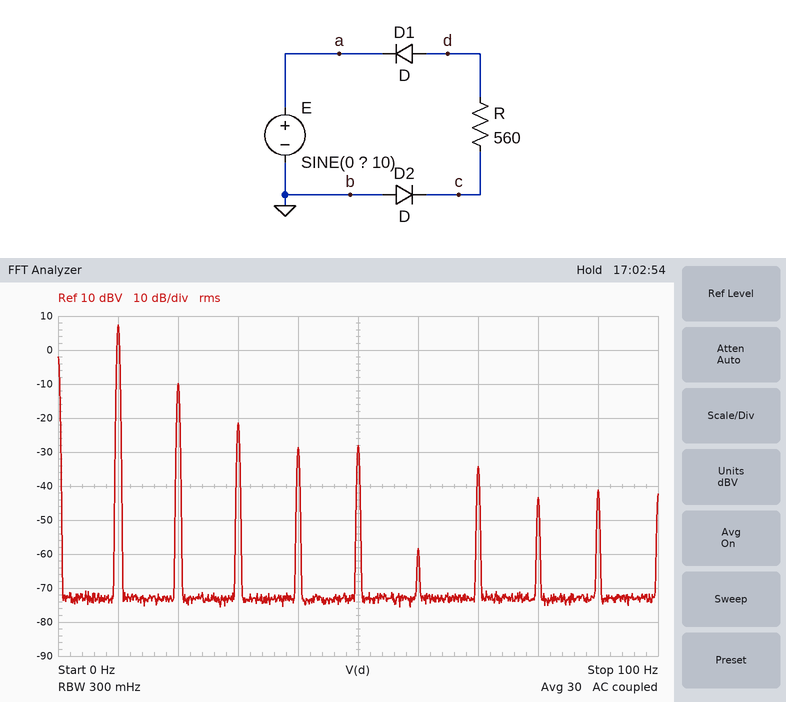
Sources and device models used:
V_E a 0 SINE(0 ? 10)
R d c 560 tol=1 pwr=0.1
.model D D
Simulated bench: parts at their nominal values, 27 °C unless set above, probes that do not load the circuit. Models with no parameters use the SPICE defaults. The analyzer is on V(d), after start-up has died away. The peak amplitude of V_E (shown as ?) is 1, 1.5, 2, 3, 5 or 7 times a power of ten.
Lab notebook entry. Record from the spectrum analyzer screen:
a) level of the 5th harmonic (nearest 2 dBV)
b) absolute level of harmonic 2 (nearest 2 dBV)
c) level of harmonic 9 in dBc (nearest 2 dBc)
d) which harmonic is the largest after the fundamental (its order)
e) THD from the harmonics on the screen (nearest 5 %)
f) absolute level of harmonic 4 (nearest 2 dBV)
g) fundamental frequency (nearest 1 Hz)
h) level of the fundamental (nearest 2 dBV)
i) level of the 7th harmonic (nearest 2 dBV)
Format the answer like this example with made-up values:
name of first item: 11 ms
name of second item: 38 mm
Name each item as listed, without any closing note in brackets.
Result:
level of the 5th harmonic: -28 dBV
absolute level of harmonic 2: -10 dBV
level of harmonic 9 in dBc: -48 dBc
which harmonic is the largest after the fundamental: 2
THD from the harmonics on the screen: 15 %
absolute level of harmonic 4: -28 dBV
fundamental frequency: 10 Hz
level of the fundamental: 8 dBV
level of the 7th harmonic: -34 dBV
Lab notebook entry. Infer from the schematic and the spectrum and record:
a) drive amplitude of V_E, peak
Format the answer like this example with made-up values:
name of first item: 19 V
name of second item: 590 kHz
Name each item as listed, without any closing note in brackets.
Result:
drive amplitude of V_E, peak: 5 V
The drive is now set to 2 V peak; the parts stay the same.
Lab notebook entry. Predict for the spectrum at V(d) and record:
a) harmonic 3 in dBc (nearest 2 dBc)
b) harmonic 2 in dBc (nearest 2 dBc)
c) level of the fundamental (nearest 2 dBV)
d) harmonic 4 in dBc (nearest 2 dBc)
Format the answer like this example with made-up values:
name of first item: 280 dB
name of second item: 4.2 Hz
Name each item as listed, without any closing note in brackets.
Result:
harmonic 3 in dBc: -26 dBc
harmonic 2 in dBc: -22 dBc
level of the fundamental: -2 dBV
harmonic 4 in dBc: -34 dBc
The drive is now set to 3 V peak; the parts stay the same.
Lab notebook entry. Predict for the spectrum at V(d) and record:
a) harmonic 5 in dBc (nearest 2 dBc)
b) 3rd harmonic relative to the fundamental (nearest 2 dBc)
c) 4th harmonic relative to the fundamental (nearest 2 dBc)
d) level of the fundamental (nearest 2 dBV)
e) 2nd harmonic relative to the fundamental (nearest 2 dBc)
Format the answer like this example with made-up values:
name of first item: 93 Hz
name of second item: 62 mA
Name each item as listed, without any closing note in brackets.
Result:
harmonic 5 in dBc: -36 dBc
3rd harmonic relative to the fundamental: -26 dBc
4th harmonic relative to the fundamental: -54 dBc
level of the fundamental: 2 dBV
2nd harmonic relative to the fundamental: -18 dBc
